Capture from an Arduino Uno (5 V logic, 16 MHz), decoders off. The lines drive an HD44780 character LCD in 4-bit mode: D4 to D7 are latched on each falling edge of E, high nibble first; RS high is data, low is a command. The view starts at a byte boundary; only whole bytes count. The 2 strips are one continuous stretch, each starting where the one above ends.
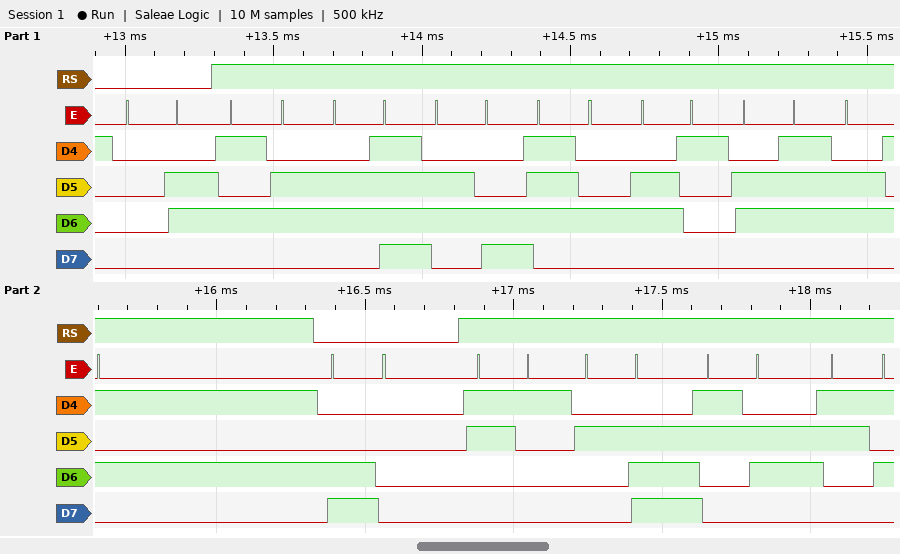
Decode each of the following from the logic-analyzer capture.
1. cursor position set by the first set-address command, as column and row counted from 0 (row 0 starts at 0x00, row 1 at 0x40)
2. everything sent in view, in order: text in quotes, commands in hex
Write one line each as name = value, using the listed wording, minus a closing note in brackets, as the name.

cursor position set by the first set-address command, as column and row counted from 0 = column 0, row 1
everything sent in view, in order: text in quotes, commands in hex = 0x06 "Voltage" 0xC0 "1.65"
